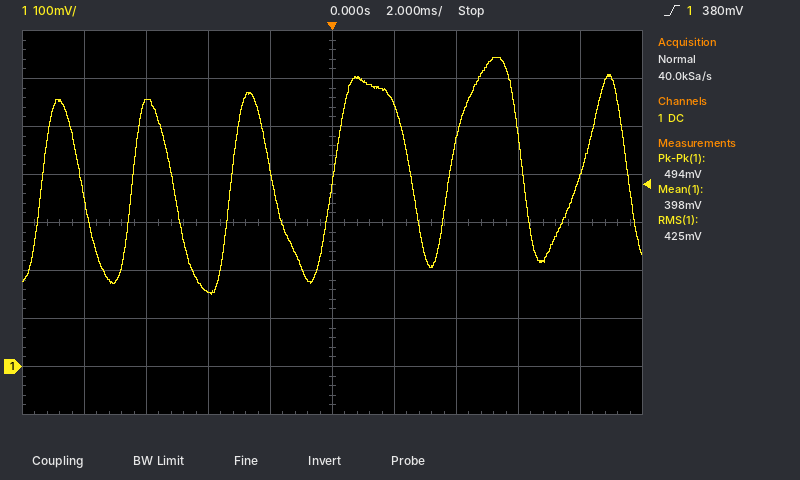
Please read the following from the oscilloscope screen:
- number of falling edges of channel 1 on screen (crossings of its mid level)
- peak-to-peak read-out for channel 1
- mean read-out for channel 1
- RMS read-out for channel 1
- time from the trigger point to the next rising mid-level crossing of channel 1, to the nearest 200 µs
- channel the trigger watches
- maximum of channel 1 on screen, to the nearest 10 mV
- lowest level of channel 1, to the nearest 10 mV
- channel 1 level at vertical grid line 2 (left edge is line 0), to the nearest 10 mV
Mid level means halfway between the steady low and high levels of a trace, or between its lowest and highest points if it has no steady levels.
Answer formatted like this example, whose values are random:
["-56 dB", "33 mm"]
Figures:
["6", "494 mV", "398 mV", "425 mV", "3.8 ms", "channel 1", "640 mV", "150 mV", "550 mV"]
